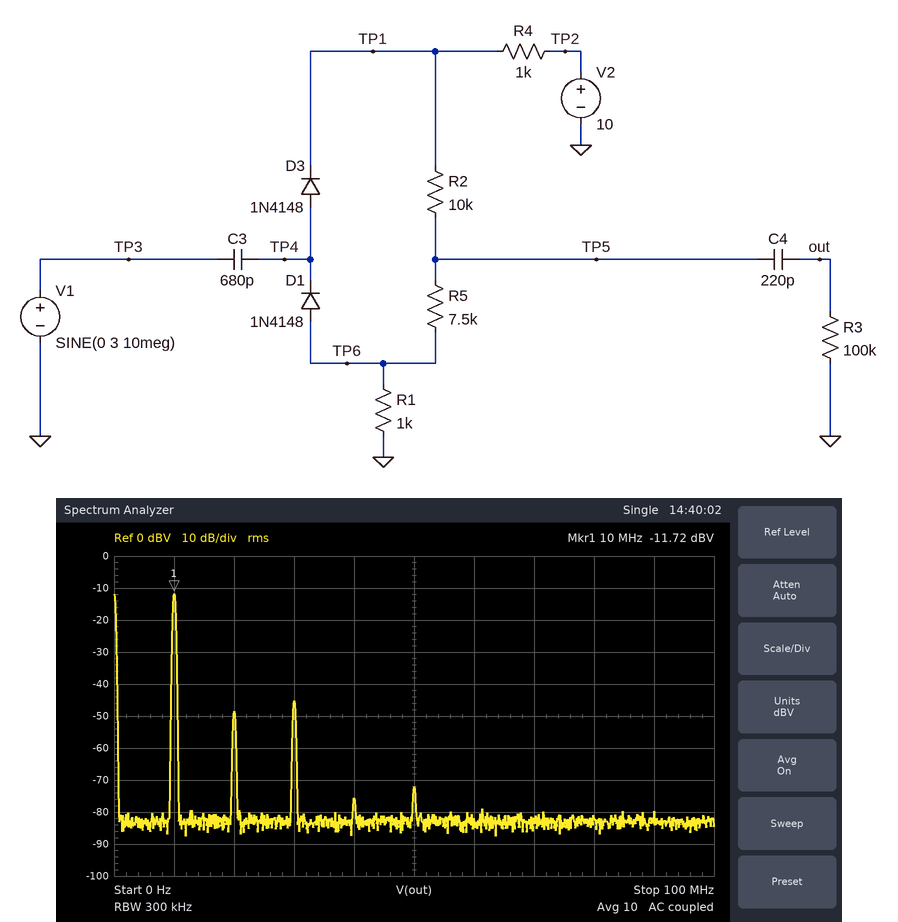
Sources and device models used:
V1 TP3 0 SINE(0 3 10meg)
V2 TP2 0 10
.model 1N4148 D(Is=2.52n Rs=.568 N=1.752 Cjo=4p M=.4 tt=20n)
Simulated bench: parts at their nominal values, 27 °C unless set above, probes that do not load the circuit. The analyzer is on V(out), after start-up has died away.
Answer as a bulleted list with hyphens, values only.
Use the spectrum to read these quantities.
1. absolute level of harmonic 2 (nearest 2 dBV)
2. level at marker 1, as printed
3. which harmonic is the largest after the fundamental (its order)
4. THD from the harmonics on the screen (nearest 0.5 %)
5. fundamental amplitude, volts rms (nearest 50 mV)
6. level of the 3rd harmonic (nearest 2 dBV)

- -48 dBV
- -11.72 dBV
- 3
- 2.5 %
- 250 mV
- -46 dBV
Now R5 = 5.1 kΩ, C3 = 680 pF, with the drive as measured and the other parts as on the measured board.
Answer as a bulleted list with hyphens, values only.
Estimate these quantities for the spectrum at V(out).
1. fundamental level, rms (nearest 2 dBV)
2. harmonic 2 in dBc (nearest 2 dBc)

- -12 dBV
- -30 dBc
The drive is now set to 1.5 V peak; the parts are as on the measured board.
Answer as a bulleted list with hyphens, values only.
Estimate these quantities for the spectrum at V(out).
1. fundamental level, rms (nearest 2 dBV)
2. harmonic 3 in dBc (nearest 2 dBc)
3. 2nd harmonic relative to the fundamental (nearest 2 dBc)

- -18 dBV
- -46 dBc
- -44 dBc
